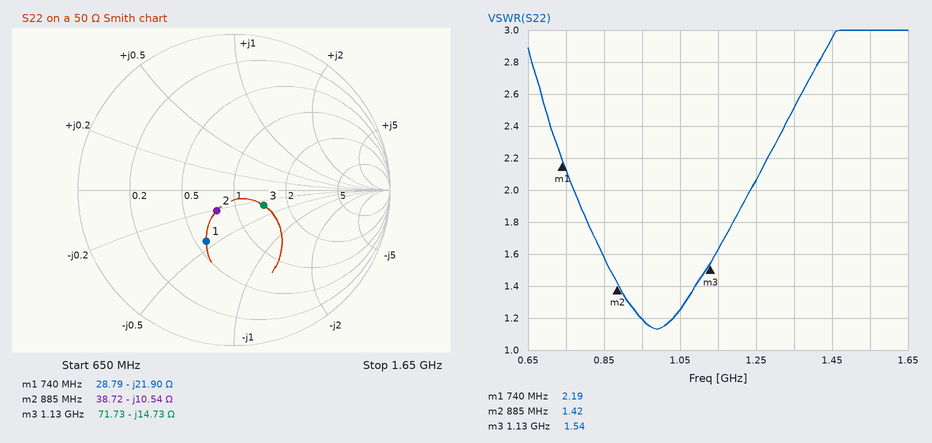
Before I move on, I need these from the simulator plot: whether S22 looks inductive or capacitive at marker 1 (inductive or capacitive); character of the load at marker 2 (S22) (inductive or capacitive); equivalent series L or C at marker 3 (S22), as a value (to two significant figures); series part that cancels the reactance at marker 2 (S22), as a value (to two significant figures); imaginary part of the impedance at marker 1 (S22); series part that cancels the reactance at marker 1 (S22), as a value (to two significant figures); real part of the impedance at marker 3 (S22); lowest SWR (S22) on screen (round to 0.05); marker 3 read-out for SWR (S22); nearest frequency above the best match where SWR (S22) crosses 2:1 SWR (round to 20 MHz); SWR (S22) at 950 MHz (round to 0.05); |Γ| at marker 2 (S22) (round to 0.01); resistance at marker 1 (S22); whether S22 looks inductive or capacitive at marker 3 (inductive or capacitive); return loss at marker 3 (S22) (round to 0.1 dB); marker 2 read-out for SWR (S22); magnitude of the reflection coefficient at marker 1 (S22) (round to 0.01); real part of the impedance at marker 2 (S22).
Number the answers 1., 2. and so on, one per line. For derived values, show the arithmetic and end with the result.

1. capacitive
2. capacitive
3. C = 1/(2π × 1.13 GHz × 14.73 Ω) ≈ 9.6 pF
4. L = 10.54 Ω/(2π × 885 MHz) ≈ 1.9 nH
5. -21.90 Ω
6. L = 21.9 Ω/(2π × 740 MHz) ≈ 4.7 nH
7. 71.73 Ω
8. 1.15
9. 1.54
10. 1.24 GHz
11. 1.20
12. 0.17
13. 28.79 Ω
14. capacitive
15. 13.4 dB
16. 1.42
17. 0.37
18. 38.72 Ω
